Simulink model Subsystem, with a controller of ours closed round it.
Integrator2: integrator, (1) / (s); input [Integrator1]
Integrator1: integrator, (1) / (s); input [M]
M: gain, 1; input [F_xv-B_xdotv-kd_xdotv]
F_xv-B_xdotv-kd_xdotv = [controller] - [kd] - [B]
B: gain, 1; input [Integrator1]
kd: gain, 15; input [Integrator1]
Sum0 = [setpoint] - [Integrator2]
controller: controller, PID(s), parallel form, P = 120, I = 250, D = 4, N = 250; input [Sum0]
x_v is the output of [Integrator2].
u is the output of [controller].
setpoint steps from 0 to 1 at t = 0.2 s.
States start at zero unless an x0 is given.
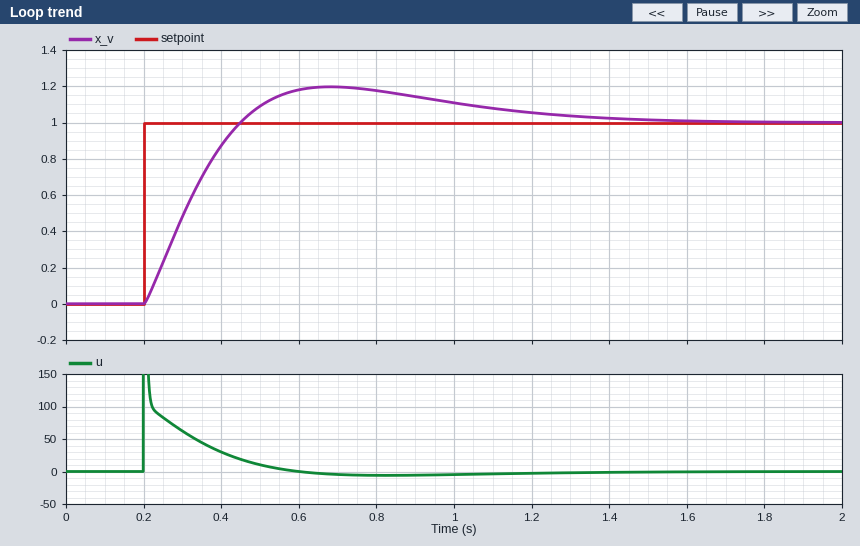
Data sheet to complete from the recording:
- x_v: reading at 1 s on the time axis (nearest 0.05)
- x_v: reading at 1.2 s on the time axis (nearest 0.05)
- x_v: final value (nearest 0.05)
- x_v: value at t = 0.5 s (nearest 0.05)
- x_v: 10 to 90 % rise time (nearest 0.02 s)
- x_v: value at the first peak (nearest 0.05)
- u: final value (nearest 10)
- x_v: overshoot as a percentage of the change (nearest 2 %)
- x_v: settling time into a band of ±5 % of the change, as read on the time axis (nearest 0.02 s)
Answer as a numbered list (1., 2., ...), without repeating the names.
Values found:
1. 1.10
2. 1.05
3. 1.00
4. 1.10
5. 0.18 s
6. 1.20
7. 0
8. 20 %
9. 1.22 s
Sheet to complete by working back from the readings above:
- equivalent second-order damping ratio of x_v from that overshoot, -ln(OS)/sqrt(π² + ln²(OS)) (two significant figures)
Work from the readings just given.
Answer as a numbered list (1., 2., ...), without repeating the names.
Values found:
1. 0.46
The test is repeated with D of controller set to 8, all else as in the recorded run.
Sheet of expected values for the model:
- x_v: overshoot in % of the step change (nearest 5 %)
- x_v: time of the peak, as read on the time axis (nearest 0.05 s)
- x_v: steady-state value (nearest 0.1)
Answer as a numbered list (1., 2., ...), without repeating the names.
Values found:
1. 15 %
2. 0.75 s
3. 1.0
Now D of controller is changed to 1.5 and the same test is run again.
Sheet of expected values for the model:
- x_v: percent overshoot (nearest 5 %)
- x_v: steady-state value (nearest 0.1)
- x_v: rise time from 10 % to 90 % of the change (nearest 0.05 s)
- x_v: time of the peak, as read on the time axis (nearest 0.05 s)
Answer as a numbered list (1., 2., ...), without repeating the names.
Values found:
1. 25 %
2. 1.0
3. 0.15 s
4. 0.65 s
